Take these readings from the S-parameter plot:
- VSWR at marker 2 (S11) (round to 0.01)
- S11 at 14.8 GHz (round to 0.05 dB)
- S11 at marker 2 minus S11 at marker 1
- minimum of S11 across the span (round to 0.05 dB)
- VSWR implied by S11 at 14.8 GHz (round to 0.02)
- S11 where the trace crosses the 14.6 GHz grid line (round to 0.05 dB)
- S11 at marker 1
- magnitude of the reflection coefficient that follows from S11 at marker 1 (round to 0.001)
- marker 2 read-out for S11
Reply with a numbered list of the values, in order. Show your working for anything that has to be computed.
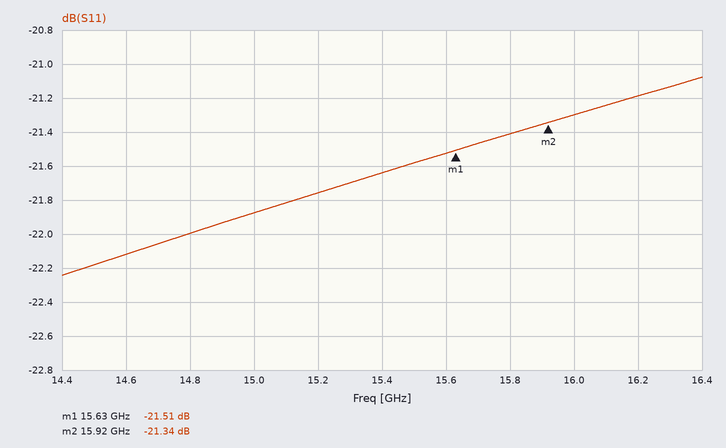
1. (1 + 0.0857)/(1 − 0.0857) ≈ 1.19
2. -22.00 dB
3. -21.34 − (-21.51) = 0.17 dB
4. -22.25 dB
5. |Γ| = 10^(-22/20) = 0.0794; VSWR = (1 + 0.0794)/(1 − 0.0794) ≈ 1.17, so 1.18 to the nearest 0.02
6. -22.10 dB
7. -21.51 dB
8. 10^(-21.51/20) ≈ 0.084
9. -21.34 dB
